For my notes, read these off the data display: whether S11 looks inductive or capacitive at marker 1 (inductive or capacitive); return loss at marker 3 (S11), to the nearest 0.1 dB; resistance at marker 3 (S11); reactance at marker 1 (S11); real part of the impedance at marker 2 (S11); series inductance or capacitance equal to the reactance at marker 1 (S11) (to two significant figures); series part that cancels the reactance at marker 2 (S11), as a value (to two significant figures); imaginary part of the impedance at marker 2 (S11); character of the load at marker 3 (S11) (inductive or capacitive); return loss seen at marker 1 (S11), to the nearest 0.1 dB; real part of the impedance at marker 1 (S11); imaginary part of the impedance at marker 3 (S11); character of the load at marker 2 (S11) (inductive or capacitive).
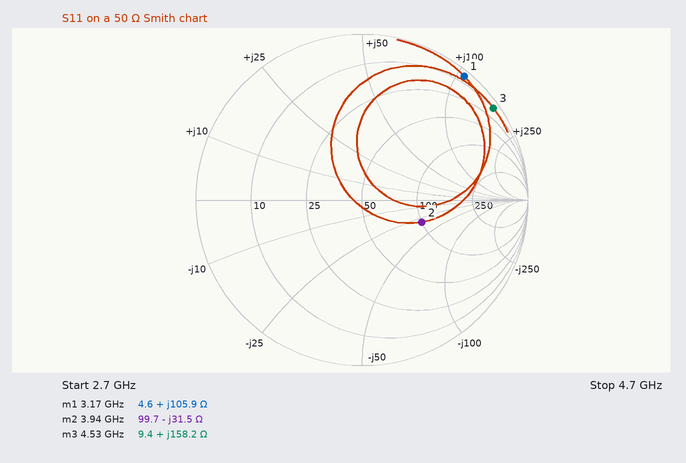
inductive
0.3 dB
9.4 Ω
+105.9 Ω
99.7 Ω
5.3 nH
1.3 nH
-31.5 Ω
inductive
0.3 dB
4.6 Ω
+158.2 Ω
capacitive
